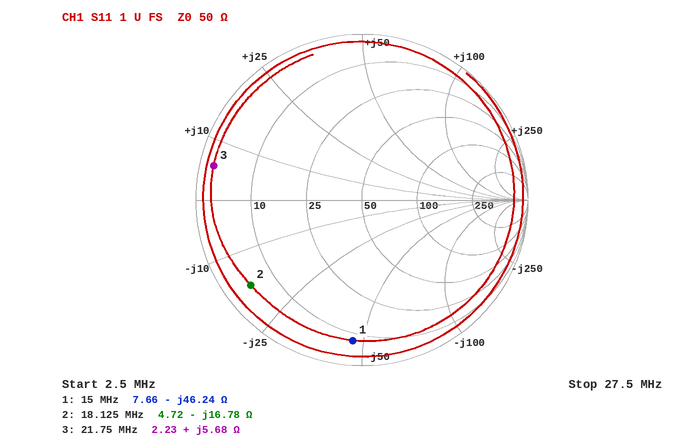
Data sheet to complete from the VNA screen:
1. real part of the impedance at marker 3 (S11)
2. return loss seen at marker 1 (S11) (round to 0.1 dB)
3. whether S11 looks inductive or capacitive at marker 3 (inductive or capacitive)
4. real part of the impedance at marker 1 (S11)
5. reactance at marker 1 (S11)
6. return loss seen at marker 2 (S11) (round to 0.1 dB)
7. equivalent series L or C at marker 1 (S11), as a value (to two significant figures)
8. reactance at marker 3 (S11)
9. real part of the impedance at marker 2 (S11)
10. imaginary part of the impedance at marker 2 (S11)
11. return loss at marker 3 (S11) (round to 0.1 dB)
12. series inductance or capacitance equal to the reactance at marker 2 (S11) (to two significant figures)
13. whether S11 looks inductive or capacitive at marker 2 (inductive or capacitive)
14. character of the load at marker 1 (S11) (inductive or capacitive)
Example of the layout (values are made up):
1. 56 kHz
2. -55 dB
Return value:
1. 2.23 Ω
2. 1.4 dB
3. inductive
4. 7.66 Ω
5. -46.24 Ω
6. 1.5 dB
7. 230 pF
8. +5.68 Ω
9. 4.72 Ω
10. -16.78 Ω
11. 0.8 dB
12. 520 pF
13. capacitive
14. capacitive
